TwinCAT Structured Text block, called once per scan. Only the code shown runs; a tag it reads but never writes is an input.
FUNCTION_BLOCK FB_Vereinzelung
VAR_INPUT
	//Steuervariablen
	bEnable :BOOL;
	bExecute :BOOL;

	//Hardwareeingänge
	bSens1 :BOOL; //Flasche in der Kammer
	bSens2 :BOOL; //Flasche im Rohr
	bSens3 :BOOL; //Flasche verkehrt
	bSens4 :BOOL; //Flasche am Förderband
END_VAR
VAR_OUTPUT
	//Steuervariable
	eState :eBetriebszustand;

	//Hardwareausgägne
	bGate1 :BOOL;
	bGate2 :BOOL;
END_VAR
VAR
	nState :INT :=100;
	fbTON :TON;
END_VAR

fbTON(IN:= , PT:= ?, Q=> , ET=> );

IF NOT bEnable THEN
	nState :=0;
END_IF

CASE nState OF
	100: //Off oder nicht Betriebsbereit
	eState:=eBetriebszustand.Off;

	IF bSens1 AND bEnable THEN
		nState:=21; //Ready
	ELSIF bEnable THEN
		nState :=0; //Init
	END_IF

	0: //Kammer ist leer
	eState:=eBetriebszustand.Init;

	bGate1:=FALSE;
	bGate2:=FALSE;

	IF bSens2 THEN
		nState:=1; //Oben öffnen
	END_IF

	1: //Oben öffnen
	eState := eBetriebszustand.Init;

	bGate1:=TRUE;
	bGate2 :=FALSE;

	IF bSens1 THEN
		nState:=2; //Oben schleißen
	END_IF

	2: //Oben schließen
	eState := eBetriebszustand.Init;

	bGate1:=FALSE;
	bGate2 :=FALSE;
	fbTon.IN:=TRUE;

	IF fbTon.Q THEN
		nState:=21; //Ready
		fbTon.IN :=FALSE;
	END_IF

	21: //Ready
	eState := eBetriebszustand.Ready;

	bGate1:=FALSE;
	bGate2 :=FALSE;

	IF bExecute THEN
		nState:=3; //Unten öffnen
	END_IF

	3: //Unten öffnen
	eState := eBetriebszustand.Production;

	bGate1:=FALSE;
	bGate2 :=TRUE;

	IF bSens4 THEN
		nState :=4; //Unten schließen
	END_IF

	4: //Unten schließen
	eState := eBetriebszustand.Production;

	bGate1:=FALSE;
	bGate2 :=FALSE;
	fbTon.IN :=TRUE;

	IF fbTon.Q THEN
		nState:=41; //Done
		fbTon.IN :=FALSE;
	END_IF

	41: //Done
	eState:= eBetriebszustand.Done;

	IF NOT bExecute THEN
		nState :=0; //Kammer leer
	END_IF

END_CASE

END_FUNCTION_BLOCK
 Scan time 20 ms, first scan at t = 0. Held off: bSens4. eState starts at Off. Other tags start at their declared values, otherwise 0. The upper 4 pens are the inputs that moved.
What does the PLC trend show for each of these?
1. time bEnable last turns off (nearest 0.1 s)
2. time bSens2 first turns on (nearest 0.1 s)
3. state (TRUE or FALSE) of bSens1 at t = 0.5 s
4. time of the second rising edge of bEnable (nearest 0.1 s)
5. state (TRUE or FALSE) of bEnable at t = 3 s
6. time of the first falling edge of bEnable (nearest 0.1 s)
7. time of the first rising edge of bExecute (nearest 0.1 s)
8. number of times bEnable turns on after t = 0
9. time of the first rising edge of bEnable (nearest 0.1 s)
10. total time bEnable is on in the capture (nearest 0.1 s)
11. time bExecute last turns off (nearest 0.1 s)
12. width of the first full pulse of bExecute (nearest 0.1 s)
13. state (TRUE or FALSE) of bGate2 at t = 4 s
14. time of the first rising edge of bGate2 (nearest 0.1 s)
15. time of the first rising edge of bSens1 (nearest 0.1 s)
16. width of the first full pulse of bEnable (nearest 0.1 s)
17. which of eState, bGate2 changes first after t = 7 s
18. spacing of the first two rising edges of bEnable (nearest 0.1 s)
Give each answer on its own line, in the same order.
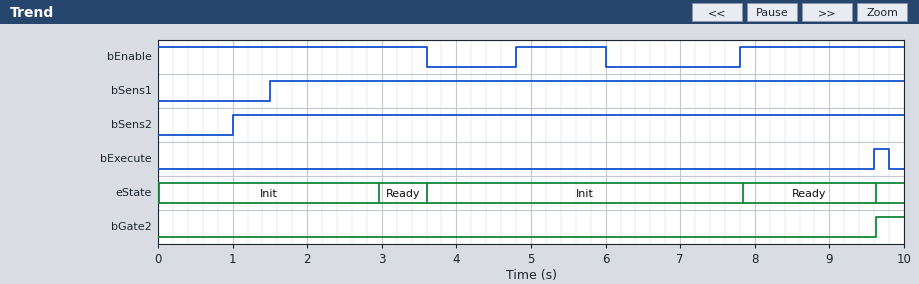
6.0 s
1.0 s
FALSE
7.8 s
TRUE
3.6 s
9.6 s
2
4.8 s
7.0 s
9.8 s
0.2 s
FALSE
9.6 s
1.5 s
1.2 s
eState
3.0 s
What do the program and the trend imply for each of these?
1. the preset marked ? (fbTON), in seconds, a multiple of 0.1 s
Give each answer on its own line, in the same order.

1.4 s
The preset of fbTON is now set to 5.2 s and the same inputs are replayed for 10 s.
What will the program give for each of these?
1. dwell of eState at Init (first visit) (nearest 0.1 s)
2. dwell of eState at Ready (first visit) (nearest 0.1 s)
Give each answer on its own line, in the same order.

7.8 s
1.8 s
